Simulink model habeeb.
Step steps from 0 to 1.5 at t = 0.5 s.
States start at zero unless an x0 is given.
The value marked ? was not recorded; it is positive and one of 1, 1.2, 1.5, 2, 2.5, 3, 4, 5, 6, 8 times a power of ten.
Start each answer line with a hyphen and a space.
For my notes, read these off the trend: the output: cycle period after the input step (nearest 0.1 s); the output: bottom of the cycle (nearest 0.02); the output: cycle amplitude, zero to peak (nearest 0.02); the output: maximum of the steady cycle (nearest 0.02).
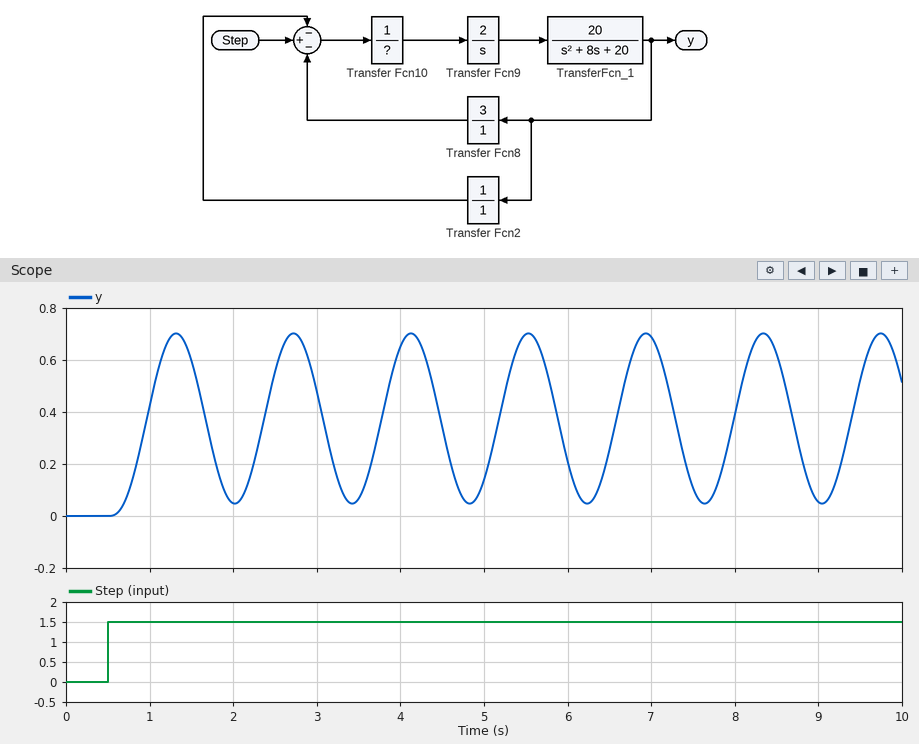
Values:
- 1.4 s
- 0.04
- 0.32
- 0.70
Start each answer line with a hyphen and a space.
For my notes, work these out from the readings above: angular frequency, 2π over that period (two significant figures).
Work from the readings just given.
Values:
- 4.5 rad/s
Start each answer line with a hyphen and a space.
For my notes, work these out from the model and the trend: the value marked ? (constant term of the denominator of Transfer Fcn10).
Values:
- 1
